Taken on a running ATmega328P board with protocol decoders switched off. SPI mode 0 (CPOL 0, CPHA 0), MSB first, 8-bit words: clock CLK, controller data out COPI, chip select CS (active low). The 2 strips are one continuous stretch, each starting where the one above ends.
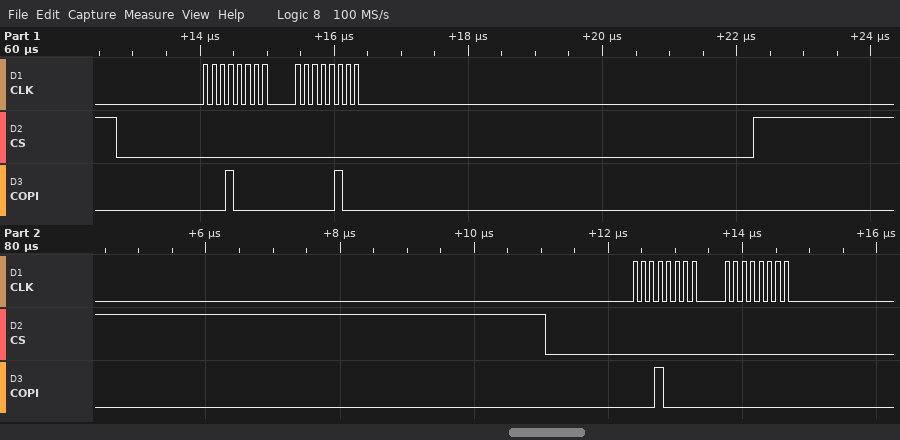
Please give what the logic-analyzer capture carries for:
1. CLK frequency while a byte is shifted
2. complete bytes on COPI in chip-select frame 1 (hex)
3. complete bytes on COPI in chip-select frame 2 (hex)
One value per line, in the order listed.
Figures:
8 MHz
10 04
10 00
